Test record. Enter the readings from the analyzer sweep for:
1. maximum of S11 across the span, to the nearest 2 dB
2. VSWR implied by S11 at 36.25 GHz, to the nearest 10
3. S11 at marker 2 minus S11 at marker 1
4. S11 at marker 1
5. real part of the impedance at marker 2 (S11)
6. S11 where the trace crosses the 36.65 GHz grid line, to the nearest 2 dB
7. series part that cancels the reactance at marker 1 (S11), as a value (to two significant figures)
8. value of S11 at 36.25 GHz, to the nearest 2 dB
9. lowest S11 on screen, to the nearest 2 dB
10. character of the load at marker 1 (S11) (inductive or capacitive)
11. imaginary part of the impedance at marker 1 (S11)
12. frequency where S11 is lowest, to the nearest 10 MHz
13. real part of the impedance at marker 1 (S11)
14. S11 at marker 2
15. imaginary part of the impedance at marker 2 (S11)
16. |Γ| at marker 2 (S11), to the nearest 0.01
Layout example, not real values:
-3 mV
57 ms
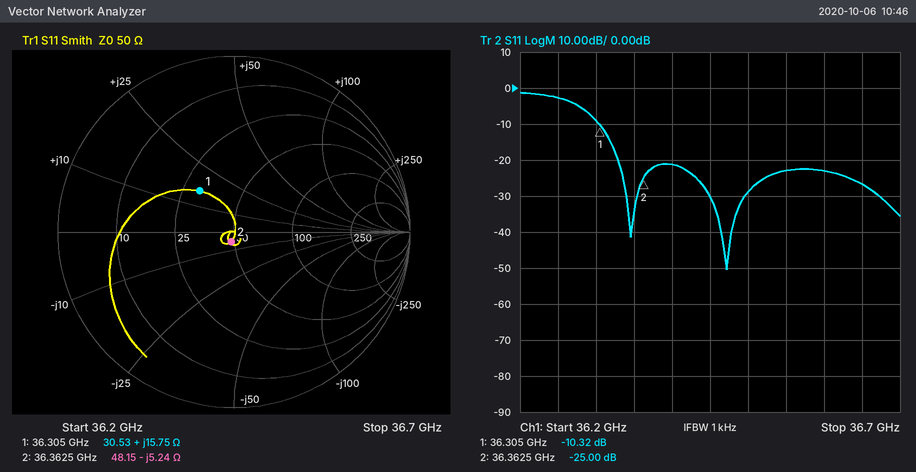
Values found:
-2 dB
10
-14.68 dB
-10.32 dB
48.15 Ω
-26 dB
280 fF
-2 dB
-50 dB
inductive
+15.75 Ω
36.47 GHz
30.53 Ω
-25.00 dB
-5.24 Ω
0.06
